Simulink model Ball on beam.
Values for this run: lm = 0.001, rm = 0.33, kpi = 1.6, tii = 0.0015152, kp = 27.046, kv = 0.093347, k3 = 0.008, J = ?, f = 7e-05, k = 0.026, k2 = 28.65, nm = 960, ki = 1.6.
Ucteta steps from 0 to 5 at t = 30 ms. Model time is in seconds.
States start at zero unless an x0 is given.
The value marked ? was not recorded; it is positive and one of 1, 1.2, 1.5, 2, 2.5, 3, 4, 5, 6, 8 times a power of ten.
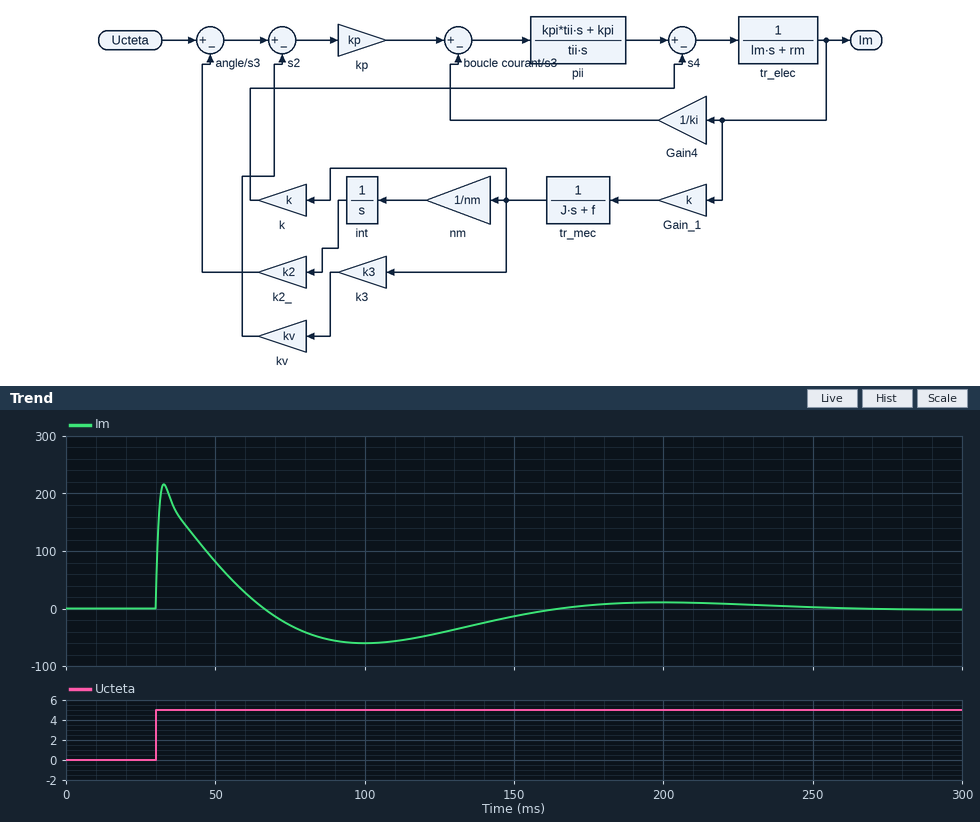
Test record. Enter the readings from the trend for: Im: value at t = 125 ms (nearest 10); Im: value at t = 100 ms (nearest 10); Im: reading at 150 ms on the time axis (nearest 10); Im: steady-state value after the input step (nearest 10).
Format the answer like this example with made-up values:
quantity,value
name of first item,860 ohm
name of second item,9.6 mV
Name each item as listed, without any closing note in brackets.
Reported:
quantity,value
Im: value at t = 125 ms,-40
Im: value at t = 100 ms,-60
Im: reading at 150 ms on the time axis,-10
Im: steady-state value after the input step,0
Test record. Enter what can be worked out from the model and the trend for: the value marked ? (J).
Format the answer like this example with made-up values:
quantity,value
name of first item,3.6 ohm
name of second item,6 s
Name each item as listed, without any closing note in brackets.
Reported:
quantity,value
the value marked ?,2.5e-05
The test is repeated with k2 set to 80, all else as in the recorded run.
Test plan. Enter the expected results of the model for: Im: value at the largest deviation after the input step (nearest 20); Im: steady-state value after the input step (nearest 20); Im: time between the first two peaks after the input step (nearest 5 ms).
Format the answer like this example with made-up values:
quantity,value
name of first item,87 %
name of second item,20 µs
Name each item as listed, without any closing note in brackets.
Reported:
quantity,value
Im: value at the largest deviation after the input step,220
Im: steady-state value after the input step,0
Im: time between the first two peaks after the input step,95 ms
